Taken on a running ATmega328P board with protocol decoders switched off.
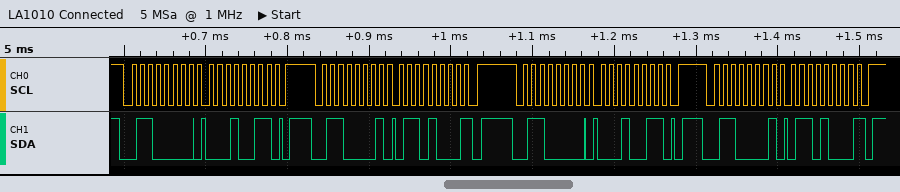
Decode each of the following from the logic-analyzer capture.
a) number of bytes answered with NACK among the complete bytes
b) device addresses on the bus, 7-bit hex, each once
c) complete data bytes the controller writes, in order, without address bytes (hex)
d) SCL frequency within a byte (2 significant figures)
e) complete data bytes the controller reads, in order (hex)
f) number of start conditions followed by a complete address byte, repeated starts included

2
0x30
13 13
100 kHz
68 68
4
